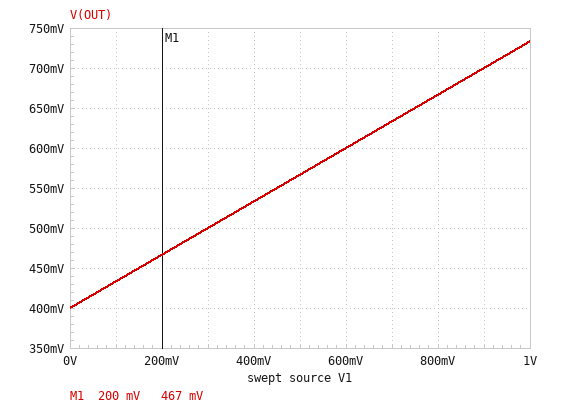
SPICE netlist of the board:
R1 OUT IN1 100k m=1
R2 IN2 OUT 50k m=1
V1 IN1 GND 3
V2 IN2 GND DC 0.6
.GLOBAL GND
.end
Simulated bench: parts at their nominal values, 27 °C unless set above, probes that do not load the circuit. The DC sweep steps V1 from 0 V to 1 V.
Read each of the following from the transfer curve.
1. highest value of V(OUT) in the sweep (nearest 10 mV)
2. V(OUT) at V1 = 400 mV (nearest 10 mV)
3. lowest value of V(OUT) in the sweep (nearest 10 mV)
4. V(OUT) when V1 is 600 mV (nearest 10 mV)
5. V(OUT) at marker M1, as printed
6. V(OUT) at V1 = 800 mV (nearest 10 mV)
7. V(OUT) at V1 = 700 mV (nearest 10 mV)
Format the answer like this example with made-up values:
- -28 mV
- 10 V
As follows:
- 730 mV
- 530 mV
- 400 mV
- 600 mV
- 467 mV
- 670 mV
- 630 mV
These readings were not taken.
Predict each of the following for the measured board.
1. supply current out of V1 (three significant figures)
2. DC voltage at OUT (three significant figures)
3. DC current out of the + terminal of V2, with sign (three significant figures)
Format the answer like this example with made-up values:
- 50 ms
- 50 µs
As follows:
- 16.0 µA
- 1.40 V
- -16.0 µA
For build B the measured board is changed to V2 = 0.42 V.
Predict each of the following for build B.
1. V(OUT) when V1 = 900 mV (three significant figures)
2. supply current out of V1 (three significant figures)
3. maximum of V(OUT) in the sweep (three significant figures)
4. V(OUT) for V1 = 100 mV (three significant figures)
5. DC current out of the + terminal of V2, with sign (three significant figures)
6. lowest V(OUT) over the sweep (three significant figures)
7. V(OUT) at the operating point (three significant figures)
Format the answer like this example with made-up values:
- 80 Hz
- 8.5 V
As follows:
- 580 mV
- 17.2 µA
- 613 mV
- 313 mV
- -17.2 µA
- 280 mV
- 1.28 V
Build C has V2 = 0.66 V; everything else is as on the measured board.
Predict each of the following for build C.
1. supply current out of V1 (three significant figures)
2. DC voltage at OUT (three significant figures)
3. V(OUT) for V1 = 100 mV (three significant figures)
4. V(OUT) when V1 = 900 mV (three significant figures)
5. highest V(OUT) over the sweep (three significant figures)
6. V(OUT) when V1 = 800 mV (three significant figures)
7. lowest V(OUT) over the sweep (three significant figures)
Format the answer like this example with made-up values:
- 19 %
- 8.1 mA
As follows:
- 15.6 µA
- 1.44 V
- 473 mV
- 740 mV
- 773 mV
- 707 mV
- 440 mV
